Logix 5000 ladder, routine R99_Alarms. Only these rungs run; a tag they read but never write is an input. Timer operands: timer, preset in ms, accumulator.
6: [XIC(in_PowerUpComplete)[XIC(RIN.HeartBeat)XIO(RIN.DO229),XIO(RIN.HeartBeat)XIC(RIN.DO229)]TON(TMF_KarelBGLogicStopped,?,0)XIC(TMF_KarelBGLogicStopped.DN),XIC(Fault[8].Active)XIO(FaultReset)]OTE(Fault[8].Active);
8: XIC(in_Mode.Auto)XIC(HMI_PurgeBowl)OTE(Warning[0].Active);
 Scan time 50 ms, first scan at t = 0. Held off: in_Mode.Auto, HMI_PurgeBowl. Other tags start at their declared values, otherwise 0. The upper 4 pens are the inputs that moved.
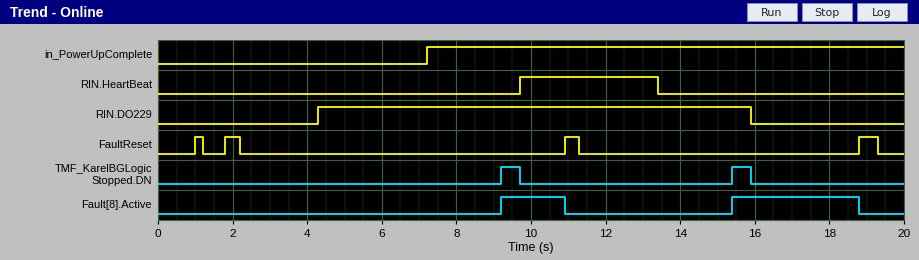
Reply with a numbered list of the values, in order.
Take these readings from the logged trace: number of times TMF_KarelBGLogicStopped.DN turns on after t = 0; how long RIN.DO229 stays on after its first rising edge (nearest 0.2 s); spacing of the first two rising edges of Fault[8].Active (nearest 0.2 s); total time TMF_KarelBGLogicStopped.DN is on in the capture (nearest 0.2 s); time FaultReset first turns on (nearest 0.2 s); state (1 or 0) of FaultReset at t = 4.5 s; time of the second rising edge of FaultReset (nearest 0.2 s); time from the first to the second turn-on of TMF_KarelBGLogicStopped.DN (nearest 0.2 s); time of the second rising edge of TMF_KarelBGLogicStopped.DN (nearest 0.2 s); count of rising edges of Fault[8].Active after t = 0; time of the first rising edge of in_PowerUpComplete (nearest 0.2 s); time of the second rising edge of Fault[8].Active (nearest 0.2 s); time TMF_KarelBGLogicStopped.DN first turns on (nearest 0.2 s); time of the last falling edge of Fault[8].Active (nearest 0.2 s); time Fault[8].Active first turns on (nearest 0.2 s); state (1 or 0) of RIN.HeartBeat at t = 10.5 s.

1. 2
2. 11.6 s
3. 6.2 s
4. 1.0 s
5. 1.0 s
6. 0
7. 1.8 s
8. 6.2 s
9. 15.4 s
10. 2
11. 7.2 s
12. 15.4 s
13. 9.2 s
14. 18.8 s
15. 9.2 s
16. 1
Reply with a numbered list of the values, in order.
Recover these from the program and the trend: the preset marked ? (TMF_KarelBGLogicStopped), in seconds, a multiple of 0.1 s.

1. 2.0 s
